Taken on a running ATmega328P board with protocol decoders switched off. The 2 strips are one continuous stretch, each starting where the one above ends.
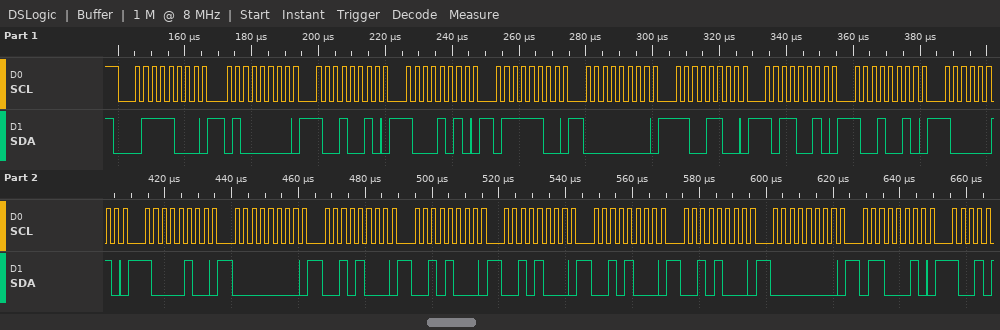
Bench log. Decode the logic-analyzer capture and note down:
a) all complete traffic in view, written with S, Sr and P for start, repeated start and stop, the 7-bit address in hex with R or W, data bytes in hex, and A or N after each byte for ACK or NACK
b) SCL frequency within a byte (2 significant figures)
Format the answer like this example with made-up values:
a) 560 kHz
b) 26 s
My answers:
a) S 3CW A 40 A 92 A 8A A 7C A 00 A CC A B2 A 92 A 82 A 84 A 00 A 28 A 28 A 28 A 28 A 28 A 00 A 62 A
b) 400 kHz
